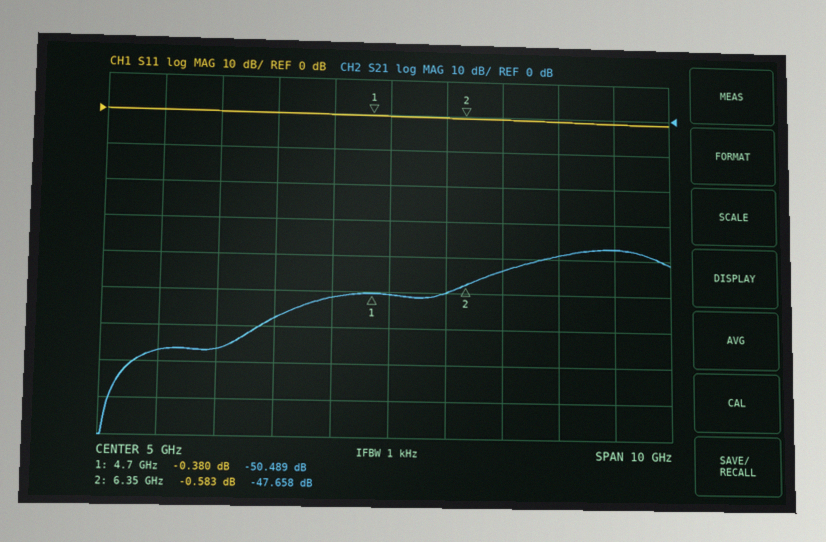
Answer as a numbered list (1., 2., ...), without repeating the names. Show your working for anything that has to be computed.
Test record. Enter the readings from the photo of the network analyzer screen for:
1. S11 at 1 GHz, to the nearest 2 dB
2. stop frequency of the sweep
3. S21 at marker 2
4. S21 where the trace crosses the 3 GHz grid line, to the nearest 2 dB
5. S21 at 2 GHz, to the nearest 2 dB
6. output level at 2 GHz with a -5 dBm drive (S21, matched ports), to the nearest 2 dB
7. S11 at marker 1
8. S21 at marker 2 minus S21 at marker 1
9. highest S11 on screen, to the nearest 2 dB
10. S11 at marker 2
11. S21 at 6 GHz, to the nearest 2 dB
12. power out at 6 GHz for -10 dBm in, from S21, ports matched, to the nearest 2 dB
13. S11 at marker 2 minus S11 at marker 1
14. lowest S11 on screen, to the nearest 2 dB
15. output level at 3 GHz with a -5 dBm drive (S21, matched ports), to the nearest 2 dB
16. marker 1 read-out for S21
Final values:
1. 0 dB
2. 10 GHz
3. -47.658 dB
4. -58 dB
5. -66 dB
6. -5 dBm + (-66 dB) = -72 dBm
7. -0.380 dB
8. -47.658 − (-50.489) = 2.831 dB
9. 0 dB
10. -0.583 dB
11. -50 dB
12. -10 dBm + (-50 dB) = -60 dBm
13. -0.583 − (-0.38) = -0.203 dB
14. -2 dB
15. -5 dBm + (-58 dB) = -62 dBm
16. -50.489 dB
